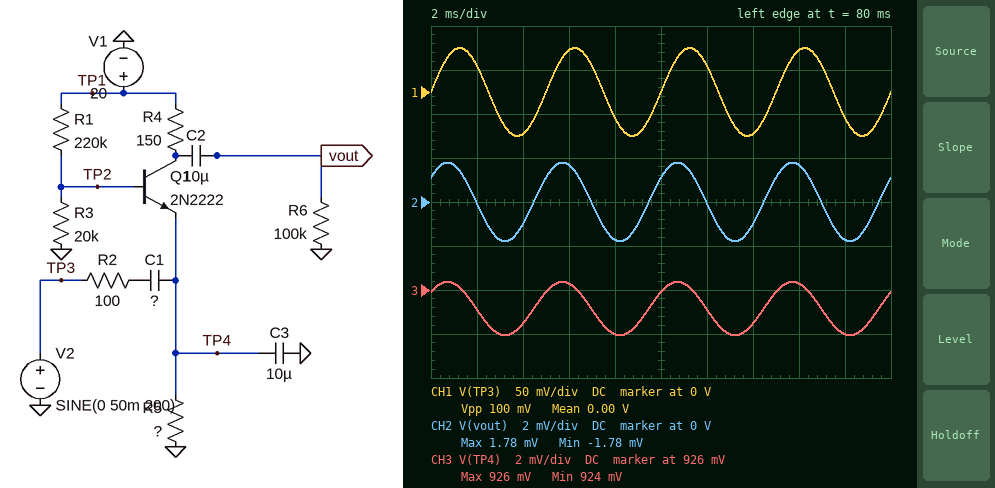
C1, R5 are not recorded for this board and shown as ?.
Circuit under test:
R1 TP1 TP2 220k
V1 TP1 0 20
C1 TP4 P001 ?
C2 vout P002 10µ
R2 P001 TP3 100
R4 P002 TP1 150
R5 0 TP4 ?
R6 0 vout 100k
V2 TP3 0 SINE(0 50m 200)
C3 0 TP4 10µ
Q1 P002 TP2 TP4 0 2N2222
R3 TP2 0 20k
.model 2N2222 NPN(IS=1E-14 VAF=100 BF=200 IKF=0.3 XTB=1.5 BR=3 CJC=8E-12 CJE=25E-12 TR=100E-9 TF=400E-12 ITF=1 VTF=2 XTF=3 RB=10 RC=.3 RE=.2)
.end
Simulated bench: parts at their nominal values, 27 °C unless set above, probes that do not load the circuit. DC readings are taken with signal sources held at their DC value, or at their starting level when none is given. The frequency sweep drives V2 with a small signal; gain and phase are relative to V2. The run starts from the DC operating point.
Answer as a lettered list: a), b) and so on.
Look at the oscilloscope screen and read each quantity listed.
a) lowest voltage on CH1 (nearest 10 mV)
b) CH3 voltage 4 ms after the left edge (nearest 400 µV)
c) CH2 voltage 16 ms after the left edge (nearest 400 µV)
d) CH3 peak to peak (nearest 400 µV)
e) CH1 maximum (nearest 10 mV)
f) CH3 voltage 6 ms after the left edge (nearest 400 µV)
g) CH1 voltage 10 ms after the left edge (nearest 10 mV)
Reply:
a) -50 mV
b) 924.4 mV
c) 1.6 mV
d) 2.4 mV
e) 50 mV
f) 926.4 mV
g) 0 V
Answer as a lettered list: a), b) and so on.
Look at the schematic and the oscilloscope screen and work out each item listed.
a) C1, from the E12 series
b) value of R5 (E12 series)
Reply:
a) 330 nF
b) 820 Ω
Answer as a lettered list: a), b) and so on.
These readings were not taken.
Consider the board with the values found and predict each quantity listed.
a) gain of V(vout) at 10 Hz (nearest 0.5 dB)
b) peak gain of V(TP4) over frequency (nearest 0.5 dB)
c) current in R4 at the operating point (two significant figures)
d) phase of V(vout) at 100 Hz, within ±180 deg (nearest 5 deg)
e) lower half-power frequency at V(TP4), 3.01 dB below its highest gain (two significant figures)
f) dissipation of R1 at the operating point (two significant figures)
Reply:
a) -51.0 dB
b) -30.0 dB
c) 1.1 mA
d) 60 deg
e) 160 Hz
f) 1.5 mW
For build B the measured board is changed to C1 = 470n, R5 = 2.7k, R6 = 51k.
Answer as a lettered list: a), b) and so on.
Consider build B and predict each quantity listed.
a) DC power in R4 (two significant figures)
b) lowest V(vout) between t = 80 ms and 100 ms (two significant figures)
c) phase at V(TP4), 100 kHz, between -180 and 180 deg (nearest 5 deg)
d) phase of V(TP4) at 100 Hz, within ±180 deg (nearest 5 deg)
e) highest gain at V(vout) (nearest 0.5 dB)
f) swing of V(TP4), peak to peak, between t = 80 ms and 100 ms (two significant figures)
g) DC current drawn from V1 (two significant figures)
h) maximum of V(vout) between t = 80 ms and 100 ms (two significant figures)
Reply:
a) 21 µW
b) -2.0 mV
c) -90 deg
d) 45 deg
e) -27.0 dB
f) 3.9 mV
g) 460 µA
h) 2.0 mV
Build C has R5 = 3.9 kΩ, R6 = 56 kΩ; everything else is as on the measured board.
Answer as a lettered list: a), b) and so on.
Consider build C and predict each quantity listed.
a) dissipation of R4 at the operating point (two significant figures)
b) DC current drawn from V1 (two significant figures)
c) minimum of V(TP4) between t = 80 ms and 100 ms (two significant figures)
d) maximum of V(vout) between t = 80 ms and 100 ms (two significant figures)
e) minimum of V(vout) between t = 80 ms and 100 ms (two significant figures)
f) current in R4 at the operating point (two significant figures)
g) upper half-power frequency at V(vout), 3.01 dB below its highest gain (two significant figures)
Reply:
a) 10 µW
b) 350 µA
c) 1.0 V
d) 1.2 mV
e) -1.2 mV
f) 260 µA
g) 5.2 kHz
